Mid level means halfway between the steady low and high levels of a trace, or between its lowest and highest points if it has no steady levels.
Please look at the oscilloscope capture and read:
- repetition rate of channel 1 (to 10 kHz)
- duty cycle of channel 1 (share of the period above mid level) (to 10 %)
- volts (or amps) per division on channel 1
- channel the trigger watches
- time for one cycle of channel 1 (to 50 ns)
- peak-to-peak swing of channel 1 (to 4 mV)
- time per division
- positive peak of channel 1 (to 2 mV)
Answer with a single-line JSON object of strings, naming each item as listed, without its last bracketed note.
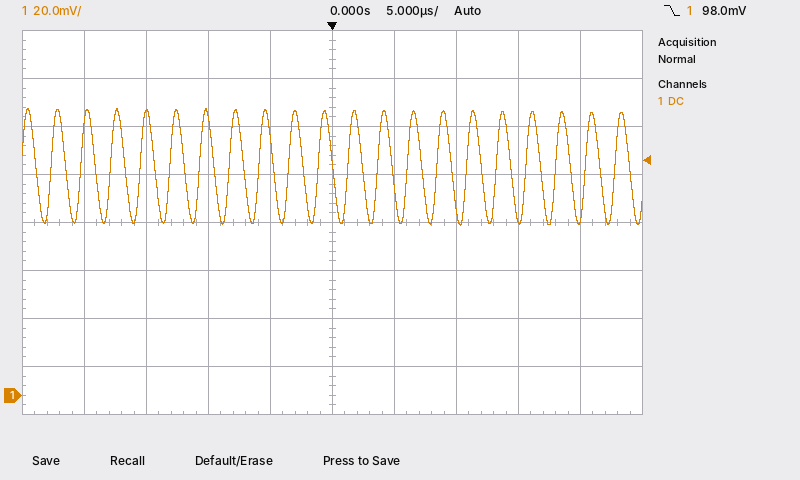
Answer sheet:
{"repetition rate of channel 1": "420 kHz", "duty cycle of channel 1 (share of the period above mid level)": "50 %", "volts (or amps) per division on channel 1": "20 mV", "channel the trigger watches": "channel 1", "time for one cycle of channel 1": "2.40 µs", "peak-to-peak swing of channel 1": "48 mV", "time per division": "5 µs", "positive peak of channel 1": "120 mV"}
